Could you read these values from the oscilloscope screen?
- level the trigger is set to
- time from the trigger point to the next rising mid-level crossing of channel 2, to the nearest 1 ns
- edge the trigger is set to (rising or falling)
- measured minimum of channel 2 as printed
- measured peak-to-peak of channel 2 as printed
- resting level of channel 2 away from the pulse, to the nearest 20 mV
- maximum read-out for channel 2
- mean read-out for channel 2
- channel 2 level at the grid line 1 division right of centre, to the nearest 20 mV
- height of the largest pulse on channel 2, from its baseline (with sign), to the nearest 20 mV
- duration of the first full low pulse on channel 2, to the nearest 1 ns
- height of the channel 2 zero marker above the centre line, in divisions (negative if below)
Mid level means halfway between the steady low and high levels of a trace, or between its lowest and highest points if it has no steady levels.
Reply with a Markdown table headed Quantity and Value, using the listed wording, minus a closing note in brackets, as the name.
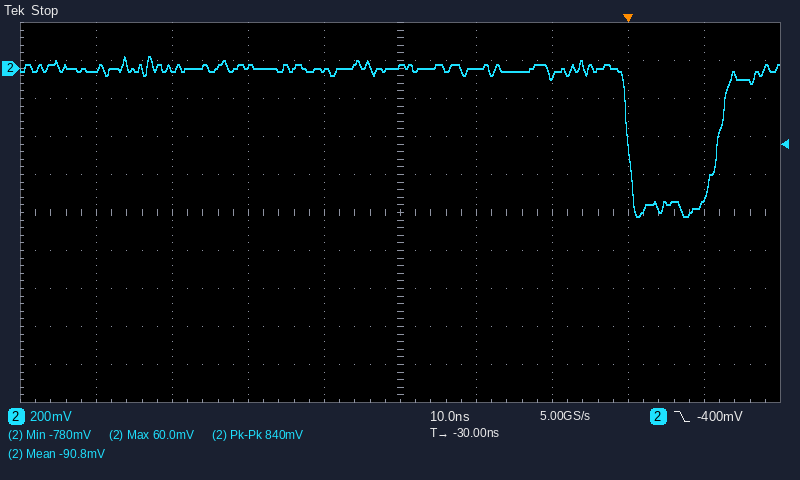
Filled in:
| Quantity | Value |
|---|---|
| level the trigger is set to | -400 mV |
| time from the trigger point to the next rising mid-level crossing of channel 2, to the nearest 1 ns | 12 ns |
| edge the trigger is set to | falling |
| measured minimum of channel 2 as printed | -780 mV |
| measured peak-to-peak of channel 2 as printed | 840 mV |
| resting level of channel 2 away from the pulse, to the nearest 20 mV | 0 mV |
| maximum read-out for channel 2 | 60.0 mV |
| mean read-out for channel 2 | -90.8 mV |
| channel 2 level at the grid line 1 division right of centre, to the nearest 20 mV | 0 mV |
| height of the largest pulse on channel 2, from its baseline (with sign), to the nearest 20 mV | -780 mV |
| duration of the first full low pulse on channel 2, to the nearest 1 ns | 12 ns |
| height of the channel 2 zero marker above the centre line, in divisions | +3.8 div |
